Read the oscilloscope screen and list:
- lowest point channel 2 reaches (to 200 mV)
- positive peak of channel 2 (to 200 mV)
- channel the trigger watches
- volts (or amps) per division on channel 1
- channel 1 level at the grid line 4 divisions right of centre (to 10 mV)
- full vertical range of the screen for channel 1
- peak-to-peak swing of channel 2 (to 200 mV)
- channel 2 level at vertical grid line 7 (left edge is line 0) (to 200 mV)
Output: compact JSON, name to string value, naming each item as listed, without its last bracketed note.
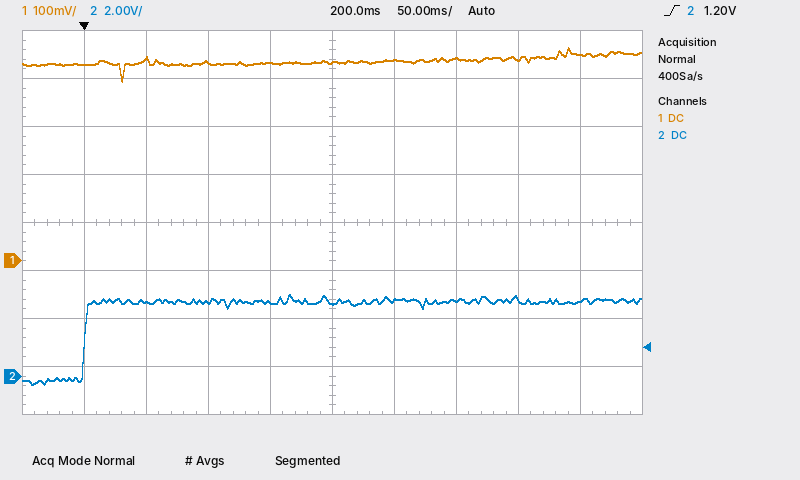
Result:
{"lowest point channel 2 reaches": "-400 mV", "positive peak of channel 2": "3.4 V", "channel the trigger watches": "channel 2", "volts (or amps) per division on channel 1": "100 mV", "channel 1 level at the grid line 4 divisions right of centre": "430 mV", "full vertical range of the screen for channel 1": "800 mV", "peak-to-peak swing of channel 2": "3.8 V", "channel 2 level at vertical grid line 7 (left edge is line 0)": "3.2 V"}
